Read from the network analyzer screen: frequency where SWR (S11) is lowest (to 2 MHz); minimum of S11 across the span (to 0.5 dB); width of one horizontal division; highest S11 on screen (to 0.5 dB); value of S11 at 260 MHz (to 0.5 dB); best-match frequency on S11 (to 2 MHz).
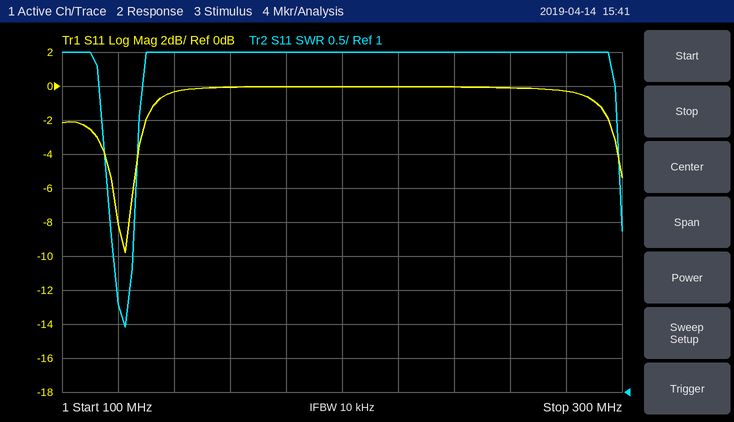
122 MHz
-10.0 dB
20 MHz
0.0 dB
0.0 dB
122 MHz
